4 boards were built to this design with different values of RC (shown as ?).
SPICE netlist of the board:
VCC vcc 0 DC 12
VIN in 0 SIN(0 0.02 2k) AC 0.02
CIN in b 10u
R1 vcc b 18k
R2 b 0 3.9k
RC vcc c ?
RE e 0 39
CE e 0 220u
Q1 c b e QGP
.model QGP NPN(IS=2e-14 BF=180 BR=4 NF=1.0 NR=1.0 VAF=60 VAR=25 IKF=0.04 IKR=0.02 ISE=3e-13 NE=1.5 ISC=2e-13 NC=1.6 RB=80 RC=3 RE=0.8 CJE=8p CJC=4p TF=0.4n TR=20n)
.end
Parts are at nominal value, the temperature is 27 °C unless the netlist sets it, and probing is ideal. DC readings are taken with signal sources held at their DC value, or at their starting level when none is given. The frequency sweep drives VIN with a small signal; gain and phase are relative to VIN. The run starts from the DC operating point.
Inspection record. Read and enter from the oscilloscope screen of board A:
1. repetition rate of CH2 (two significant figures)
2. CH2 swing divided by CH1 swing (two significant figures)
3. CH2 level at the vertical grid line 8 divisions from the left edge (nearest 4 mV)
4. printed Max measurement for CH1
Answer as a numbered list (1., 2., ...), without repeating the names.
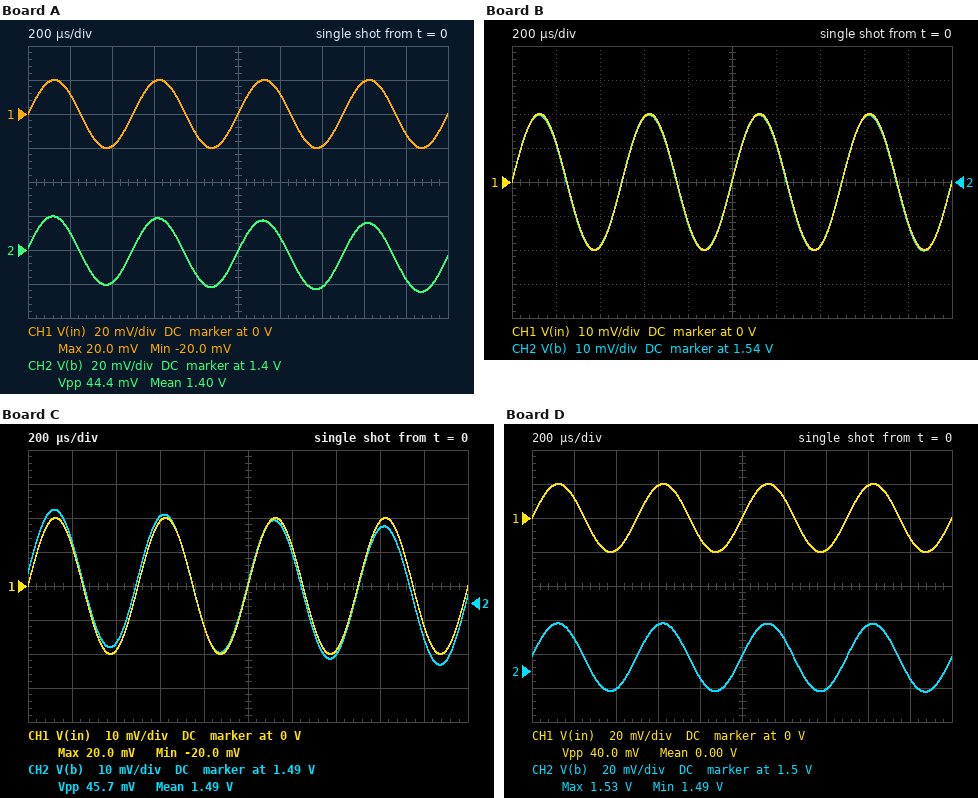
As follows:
1. 2.0 kHz
2. 1.1
3. 1.416 V
4. 20.0 mV
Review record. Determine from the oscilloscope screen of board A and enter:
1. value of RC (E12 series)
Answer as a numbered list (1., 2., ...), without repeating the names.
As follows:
1. 680 Ω
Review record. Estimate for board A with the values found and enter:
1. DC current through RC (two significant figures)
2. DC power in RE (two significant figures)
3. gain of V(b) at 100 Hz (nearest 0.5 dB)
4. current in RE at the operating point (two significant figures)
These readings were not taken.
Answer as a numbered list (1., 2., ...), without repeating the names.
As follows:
1. 16 mA
2. 11 mW
3. -6.5 dB
4. 17 mA
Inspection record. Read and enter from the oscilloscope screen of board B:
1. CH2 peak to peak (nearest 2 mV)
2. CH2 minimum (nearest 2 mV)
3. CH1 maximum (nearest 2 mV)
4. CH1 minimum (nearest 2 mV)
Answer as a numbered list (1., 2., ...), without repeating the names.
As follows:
1. 40 mV
2. 1.520 V
3. 20 mV
4. -20 mV
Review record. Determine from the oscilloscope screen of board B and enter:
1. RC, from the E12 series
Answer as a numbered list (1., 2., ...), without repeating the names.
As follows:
1. 180 Ω
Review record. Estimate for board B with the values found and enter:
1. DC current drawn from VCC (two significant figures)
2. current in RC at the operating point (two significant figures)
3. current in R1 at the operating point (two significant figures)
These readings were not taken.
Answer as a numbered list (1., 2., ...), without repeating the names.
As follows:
1. 21 mA
2. 20 mA
3. 580 µA
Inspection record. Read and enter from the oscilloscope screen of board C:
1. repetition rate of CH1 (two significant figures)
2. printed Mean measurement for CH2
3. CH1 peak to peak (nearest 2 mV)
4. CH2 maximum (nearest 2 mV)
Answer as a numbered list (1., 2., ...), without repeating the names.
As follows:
1. 2.0 kHz
2. 1.49 V
3. 40 mV
4. 1.518 V
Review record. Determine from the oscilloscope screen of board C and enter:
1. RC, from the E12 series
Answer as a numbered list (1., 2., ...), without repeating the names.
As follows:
1. 560 Ω
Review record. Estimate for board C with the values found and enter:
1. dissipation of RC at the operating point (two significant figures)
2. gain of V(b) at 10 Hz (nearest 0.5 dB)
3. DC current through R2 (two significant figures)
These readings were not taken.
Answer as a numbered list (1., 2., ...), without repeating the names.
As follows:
1. 200 mW
2. -4.5 dB
3. 380 µA
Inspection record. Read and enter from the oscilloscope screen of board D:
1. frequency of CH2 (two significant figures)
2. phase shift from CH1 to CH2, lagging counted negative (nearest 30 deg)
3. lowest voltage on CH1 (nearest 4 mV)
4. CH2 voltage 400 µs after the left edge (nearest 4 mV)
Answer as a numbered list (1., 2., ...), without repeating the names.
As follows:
1. 2.0 kHz
2. 0 deg
3. -20 mV
4. 1.488 V
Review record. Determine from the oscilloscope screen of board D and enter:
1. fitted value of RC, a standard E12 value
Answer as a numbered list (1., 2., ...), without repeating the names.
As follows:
1. 470 Ω
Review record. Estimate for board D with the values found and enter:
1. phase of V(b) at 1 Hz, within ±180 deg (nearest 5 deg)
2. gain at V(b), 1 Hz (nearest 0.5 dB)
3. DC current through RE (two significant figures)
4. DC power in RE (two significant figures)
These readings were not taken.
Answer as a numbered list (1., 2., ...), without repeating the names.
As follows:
1. 85 deg
2. -20.5 dB
3. 19 mA
4. 15 mW
